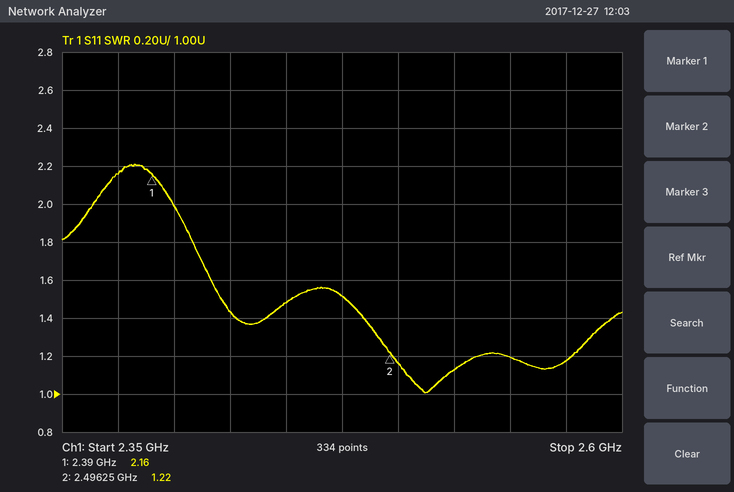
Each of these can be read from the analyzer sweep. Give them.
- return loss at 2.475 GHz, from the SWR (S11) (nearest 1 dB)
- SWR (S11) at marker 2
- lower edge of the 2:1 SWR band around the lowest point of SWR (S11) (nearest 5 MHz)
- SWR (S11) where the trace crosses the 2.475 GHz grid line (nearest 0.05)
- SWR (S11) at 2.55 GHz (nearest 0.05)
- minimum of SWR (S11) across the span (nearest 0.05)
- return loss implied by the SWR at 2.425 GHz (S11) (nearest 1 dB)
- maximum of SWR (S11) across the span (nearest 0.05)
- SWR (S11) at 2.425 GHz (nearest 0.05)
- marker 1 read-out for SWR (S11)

14 dB
1.22
2.400 GHz
1.50
1.20
1.00
15 dB
2.20
1.45
2.16
